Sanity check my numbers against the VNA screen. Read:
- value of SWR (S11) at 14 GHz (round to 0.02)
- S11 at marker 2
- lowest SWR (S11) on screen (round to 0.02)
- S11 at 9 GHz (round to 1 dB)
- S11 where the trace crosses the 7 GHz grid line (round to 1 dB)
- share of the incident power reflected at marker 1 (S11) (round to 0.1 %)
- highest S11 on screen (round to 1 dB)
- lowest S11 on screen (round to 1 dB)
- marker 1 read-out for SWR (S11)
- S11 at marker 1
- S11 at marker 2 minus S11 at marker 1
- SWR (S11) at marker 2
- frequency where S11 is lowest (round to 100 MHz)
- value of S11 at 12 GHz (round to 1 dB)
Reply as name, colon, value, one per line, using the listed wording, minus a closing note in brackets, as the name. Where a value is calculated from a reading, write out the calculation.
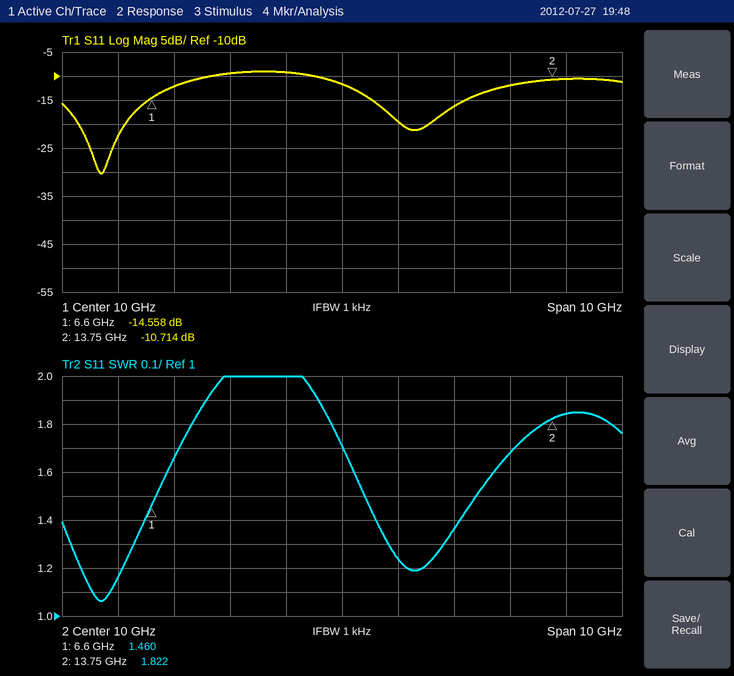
value of SWR (S11) at 14 GHz: 1.84
S11 at marker 2: -10.714 dB
lowest SWR (S11) on screen: 1.06
S11 at 9 GHz: -9 dB
S11 where the trace crosses the 7 GHz grid line: -12 dB
share of the incident power reflected at marker 1 (S11): 10^(-14.558/10) ≈ 3.5 %
highest S11 on screen: -9 dB
lowest S11 on screen: -30 dB
marker 1 read-out for SWR: 1.460
S11 at marker 1: -14.558 dB
S11 at marker 2 minus S11 at marker 1: -10.714 − (-14.558) = 3.844 dB
SWR (S11) at marker 2: 1.822
frequency where S11 is lowest: 5.7 GHz
value of S11 at 12 GHz: -16 dB
